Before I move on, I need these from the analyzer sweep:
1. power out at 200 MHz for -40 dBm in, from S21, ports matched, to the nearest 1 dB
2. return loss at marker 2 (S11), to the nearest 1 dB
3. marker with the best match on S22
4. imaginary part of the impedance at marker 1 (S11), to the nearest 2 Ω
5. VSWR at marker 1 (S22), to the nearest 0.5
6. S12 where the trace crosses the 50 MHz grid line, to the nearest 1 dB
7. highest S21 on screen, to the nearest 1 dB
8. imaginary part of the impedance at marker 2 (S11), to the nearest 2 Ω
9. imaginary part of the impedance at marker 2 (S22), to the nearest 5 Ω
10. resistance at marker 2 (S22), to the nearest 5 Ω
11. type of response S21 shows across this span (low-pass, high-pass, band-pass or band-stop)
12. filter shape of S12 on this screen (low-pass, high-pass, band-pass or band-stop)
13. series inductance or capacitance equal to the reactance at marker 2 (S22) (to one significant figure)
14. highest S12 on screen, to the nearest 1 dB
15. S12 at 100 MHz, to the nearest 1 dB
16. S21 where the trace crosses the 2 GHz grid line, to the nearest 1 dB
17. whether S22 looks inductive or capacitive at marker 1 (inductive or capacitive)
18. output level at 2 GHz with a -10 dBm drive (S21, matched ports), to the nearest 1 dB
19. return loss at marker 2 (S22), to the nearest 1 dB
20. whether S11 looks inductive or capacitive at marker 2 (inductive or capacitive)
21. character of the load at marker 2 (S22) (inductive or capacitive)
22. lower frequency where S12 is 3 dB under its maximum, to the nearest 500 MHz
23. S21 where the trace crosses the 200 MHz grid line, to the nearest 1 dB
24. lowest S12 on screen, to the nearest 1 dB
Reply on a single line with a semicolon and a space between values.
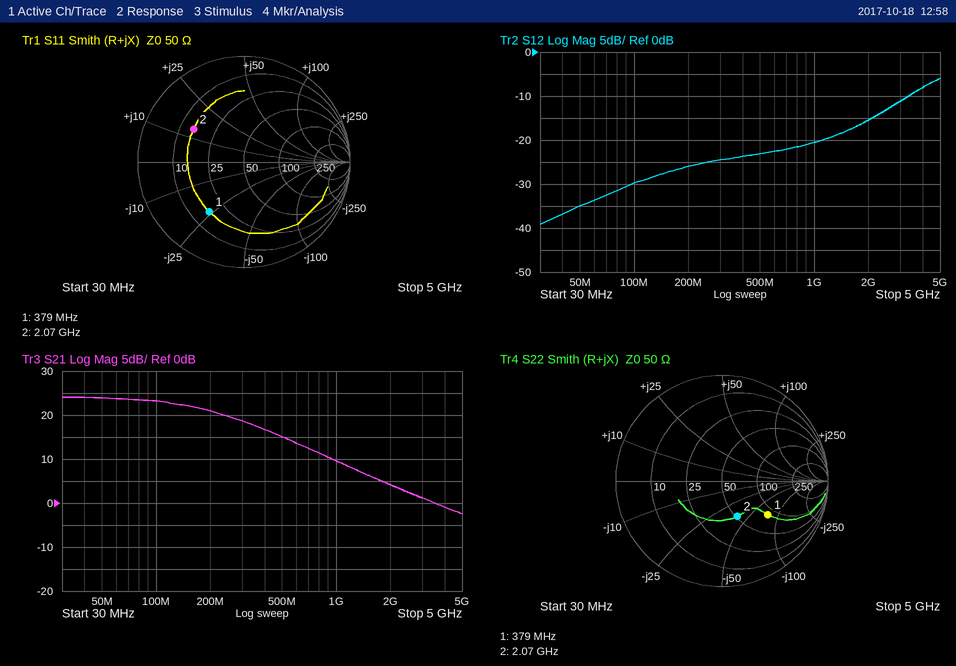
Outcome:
-19 dBm; 5 dB; marker 2; -24 Ω; 3.5; -35 dB; 24 dB; +14 Ω; -40 Ω; 50 Ω; low-pass; high-pass; 2 pF; -6 dB; -30 dB; 4 dB; capacitive; -6 dBm; 9 dB; inductive; capacitive; 3.5 GHz; 21 dB; -39 dB
